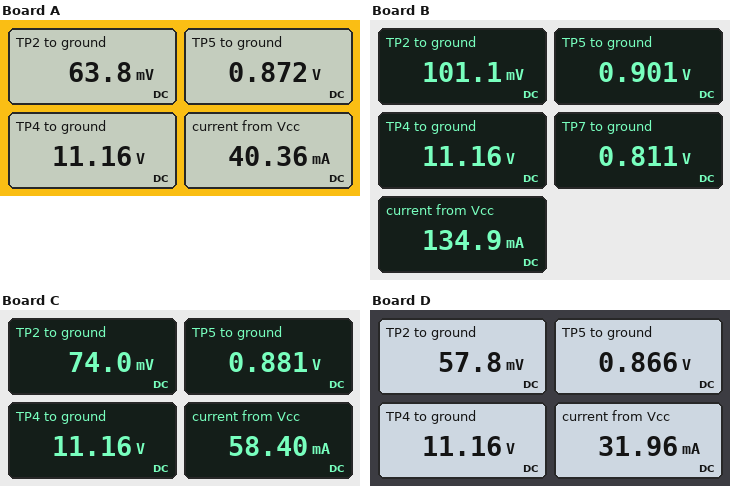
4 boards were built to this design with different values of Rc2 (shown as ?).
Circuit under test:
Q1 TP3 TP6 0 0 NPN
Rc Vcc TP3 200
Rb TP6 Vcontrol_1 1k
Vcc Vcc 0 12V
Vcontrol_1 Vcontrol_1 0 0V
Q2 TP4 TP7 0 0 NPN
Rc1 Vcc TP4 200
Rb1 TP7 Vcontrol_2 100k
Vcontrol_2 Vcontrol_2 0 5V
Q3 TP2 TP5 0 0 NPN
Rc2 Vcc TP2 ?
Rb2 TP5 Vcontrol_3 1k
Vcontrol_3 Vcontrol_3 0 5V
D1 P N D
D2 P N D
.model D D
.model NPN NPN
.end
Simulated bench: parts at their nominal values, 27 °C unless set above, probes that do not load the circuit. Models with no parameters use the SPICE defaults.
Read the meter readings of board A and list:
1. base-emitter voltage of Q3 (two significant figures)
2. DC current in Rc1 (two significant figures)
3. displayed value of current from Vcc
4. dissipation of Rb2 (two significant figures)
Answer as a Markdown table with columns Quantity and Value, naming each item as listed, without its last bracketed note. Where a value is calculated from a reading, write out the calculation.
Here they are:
| Quantity | Value |
|---|---|
| base-emitter voltage of Q3 | 872 mV = 870 mV |
| DC current in Rc1 | (12 V - 11.16 V) / 200 Ω = 4.2 mA |
| displayed value of current from Vcc | 40.36 mA |
| dissipation of Rb2 | (5 V - 872 mV)^2 / 1 kΩ = 17 mW |
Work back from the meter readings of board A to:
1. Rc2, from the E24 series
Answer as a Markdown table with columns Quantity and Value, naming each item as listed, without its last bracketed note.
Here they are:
| Quantity | Value |
|---|---|
| Rc2, from the E24 series | 330 Ω |
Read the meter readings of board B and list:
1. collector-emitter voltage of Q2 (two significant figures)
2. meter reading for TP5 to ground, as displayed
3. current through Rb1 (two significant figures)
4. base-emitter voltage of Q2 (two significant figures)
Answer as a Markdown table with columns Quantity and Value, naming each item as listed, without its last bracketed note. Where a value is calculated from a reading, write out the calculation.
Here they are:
| Quantity | Value |
|---|---|
| collector-emitter voltage of Q2 | 11.16 V = 11 V |
| meter reading for TP5 to ground, as displayed | 0.901 V |
| current through Rb1 | (5 V - 811 mV) / 100 kΩ = 42 µA |
| base-emitter voltage of Q2 | 811 mV = 810 mV |
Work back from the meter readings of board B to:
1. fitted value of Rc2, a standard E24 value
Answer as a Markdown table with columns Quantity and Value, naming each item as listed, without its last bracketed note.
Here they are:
| Quantity | Value |
|---|---|
| fitted value of Rc2, a standard E24 value | 91 Ω |
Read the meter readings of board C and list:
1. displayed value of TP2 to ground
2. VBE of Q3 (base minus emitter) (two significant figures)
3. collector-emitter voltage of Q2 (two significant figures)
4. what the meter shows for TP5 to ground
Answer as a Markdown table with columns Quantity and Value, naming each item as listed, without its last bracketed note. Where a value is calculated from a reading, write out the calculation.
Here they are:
| Quantity | Value |
|---|---|
| displayed value of TP2 to ground | 74.0 mV |
| VBE of Q3 (base minus emitter) | 881 mV = 880 mV |
| collector-emitter voltage of Q2 | 11.16 V = 11 V |
| what the meter shows for TP5 to ground | 0.881 V |
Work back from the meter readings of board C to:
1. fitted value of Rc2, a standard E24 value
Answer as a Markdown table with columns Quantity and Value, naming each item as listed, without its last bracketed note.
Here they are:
| Quantity | Value |
|---|---|
| fitted value of Rc2, a standard E24 value | 220 Ω |
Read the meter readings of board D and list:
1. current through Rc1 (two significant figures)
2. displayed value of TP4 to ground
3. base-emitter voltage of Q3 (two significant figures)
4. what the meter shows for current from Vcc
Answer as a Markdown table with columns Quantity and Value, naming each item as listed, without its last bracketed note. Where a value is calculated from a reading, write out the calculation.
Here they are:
| Quantity | Value |
|---|---|
| current through Rc1 | (12 V - 11.16 V) / 200 Ω = 4.2 mA |
| displayed value of TP4 to ground | 11.16 V |
| base-emitter voltage of Q3 | 866 mV = 870 mV |
| what the meter shows for current from Vcc | 31.96 mA |
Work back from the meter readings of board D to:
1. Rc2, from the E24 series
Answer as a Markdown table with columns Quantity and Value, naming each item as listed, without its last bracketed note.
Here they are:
| Quantity | Value |
|---|---|
| Rc2, from the E24 series | 430 Ω |
